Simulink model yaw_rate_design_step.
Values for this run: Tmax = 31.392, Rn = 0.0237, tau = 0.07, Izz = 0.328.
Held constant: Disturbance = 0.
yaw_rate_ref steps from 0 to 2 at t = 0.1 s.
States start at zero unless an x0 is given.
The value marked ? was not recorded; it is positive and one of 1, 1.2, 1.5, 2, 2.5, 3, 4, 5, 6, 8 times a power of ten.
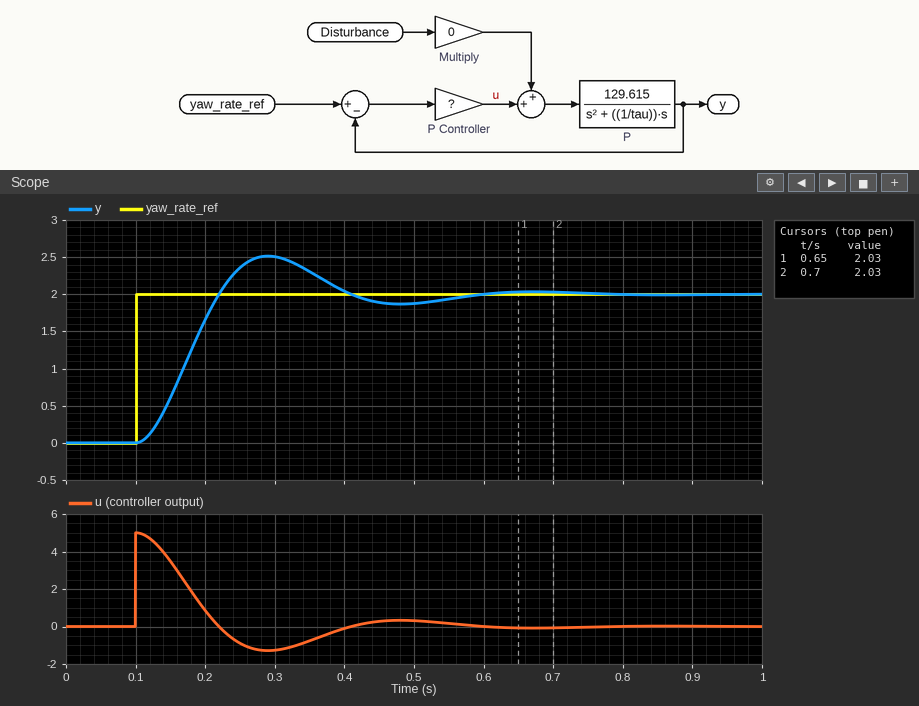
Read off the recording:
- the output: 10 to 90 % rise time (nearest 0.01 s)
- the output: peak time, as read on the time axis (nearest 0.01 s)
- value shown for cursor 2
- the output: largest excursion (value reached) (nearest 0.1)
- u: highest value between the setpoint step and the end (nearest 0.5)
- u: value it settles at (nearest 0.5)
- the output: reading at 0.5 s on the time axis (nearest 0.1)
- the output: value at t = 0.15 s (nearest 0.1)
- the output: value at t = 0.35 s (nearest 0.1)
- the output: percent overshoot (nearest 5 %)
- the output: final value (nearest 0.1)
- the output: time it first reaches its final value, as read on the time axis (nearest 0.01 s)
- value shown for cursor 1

0.08 s
0.29 s
2.03
2.5
5.0
0.0
1.9
0.6
2.3
25 %
2.0
0.22 s
2.03
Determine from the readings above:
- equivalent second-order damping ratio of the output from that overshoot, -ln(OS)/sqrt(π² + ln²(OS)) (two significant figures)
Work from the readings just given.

0.40
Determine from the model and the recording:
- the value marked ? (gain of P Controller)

2.5
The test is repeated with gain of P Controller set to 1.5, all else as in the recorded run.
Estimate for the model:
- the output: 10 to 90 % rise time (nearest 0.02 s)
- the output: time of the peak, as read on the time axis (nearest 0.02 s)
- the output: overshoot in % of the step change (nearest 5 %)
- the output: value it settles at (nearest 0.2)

0.12 s
0.36 s
15 %
2.0
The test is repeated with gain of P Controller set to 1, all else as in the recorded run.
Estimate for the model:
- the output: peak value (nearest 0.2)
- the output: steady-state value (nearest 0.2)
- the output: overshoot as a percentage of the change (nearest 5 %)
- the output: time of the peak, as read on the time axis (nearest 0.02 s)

2.2
2.0
10 %
0.46 s
